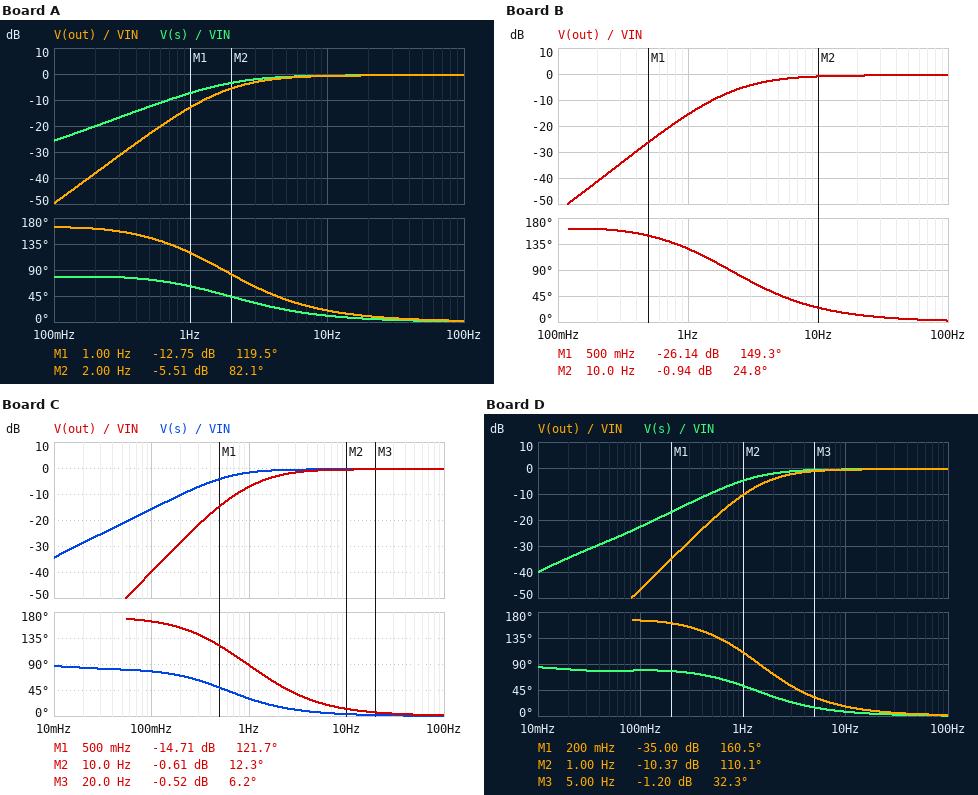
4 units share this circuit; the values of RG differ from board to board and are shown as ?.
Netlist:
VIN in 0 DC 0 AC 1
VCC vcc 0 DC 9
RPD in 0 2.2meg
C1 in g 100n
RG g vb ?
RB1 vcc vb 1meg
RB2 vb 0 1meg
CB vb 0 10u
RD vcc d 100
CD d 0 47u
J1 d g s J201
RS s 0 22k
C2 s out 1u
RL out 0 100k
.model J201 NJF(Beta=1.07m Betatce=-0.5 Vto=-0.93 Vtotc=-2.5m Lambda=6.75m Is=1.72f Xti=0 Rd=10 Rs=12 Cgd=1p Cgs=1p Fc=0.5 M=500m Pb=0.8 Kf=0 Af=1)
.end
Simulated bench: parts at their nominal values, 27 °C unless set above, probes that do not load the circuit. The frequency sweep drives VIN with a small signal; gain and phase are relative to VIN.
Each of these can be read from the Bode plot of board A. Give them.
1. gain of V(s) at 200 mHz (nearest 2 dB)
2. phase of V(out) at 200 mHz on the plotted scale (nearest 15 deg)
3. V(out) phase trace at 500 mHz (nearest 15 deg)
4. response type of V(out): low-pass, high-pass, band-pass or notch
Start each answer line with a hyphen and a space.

- -20 dB
- 165 deg
- 150 deg
- high-pass
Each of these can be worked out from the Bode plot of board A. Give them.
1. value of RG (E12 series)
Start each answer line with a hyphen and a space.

- 820 kΩ
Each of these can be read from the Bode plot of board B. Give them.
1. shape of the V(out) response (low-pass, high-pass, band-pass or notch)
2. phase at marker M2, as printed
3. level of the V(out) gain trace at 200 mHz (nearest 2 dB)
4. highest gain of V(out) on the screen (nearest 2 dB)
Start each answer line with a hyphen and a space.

- high-pass
- 24.8 deg
- -42 dB
- 0 dB
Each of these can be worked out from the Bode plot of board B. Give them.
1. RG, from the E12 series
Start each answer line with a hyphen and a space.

- 560 kΩ
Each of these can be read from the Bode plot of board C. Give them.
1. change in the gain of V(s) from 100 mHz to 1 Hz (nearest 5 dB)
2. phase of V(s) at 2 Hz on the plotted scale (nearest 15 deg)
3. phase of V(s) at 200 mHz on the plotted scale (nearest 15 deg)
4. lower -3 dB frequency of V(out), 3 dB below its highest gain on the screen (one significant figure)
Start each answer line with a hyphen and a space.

- 15 dB
- 15 deg
- 75 deg
- 2 Hz
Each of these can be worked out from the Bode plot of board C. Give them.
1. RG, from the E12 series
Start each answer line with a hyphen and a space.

- 2.7 MΩ
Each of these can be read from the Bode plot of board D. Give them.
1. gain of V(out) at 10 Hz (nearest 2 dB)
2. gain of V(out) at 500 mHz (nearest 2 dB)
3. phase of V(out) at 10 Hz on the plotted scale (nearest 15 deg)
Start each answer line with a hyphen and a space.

- 0 dB
- -20 dB
- 15 deg
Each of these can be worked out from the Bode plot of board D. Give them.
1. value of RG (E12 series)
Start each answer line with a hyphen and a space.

- 1.2 MΩ
